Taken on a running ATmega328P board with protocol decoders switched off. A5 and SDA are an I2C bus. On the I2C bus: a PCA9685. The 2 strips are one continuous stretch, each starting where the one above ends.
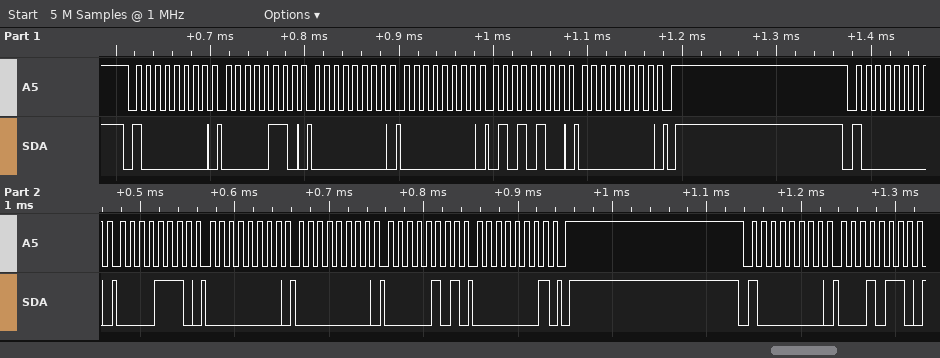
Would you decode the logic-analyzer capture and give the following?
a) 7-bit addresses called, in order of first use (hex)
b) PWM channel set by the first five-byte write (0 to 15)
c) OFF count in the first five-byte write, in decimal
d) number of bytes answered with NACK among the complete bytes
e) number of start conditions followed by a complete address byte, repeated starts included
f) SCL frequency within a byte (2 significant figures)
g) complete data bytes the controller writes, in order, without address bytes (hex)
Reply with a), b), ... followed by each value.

a) 0x40
b) 0
c) 84
d) 0
e) 3
f) 100 kHz
g) 06 00 00 54 00 0E 00 00 05 01 16
